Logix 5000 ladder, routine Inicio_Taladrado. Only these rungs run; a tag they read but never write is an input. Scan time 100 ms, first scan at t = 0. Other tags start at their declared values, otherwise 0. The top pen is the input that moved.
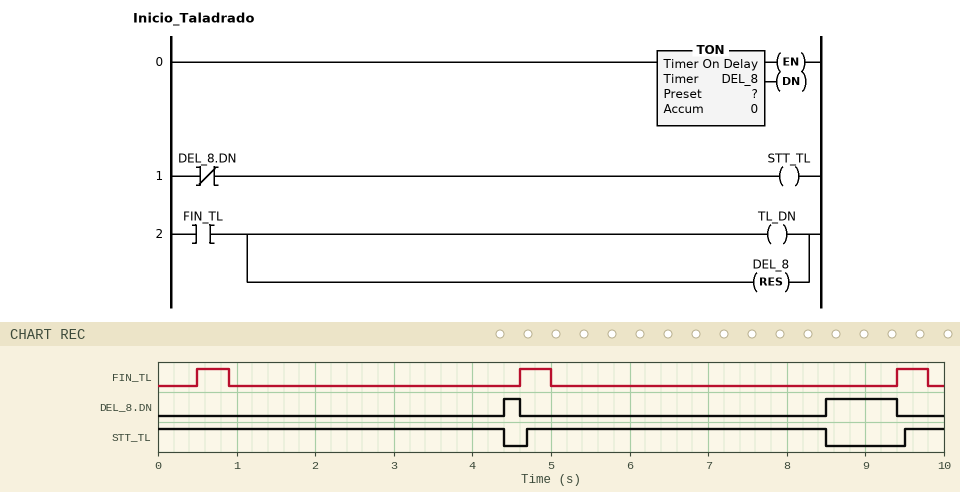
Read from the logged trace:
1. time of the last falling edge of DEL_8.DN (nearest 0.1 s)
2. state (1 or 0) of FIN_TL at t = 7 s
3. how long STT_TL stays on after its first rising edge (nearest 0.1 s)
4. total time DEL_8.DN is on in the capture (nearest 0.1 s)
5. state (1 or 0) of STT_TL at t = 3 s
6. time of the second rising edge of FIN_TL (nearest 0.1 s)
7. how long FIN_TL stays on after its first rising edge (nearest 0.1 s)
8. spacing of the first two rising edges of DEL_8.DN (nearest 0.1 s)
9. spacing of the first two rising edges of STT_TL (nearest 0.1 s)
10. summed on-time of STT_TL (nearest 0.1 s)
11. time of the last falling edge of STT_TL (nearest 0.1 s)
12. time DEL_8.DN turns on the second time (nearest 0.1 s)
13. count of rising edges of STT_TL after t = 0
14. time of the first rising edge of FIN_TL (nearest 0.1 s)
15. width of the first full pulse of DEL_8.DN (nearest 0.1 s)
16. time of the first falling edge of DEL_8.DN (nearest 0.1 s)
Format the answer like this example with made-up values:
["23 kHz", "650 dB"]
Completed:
["9.4 s", "0", "3.8 s", "1.1 s", "1", "4.6 s", "0.4 s", "4.1 s", "4.8 s", "8.7 s", "8.5 s", "8.5 s", "2", "0.5 s", "0.2 s", "4.6 s"]
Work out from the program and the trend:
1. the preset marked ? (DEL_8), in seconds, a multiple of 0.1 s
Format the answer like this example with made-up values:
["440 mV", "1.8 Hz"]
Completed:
["3.5 s"]
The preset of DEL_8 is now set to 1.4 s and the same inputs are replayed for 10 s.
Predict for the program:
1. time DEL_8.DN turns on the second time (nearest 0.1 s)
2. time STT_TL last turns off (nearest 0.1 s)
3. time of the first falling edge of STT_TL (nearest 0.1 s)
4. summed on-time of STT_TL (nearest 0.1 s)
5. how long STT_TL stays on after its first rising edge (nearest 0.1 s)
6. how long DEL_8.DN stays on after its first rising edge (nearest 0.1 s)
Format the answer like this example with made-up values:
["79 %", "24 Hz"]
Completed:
["6.4 s", "6.4 s", "2.3 s", "4.5 s", "1.7 s", "2.3 s"]
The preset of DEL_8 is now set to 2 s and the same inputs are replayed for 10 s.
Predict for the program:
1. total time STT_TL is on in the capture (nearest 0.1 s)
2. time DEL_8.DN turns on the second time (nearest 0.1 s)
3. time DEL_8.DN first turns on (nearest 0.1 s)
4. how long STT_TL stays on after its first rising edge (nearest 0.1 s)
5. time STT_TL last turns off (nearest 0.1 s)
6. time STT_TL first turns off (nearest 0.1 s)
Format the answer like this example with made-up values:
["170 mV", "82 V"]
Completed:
["5.7 s", "7.0 s", "2.9 s", "2.3 s", "7.0 s", "2.9 s"]
